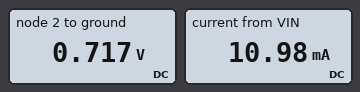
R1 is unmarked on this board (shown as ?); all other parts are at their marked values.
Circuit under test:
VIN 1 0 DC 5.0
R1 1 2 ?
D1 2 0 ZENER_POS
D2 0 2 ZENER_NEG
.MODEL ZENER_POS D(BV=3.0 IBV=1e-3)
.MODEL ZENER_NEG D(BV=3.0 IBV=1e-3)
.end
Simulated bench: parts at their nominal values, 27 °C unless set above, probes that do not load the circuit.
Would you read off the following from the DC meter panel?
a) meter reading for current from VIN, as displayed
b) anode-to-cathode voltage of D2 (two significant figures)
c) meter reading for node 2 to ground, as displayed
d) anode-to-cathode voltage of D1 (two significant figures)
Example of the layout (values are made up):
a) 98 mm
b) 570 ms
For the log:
a) 10.98 mA
b) -720 mV
c) 0.717 V
d) 720 mV
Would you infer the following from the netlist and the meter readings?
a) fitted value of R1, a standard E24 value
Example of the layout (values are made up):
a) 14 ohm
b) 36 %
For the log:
a) 390 Ω
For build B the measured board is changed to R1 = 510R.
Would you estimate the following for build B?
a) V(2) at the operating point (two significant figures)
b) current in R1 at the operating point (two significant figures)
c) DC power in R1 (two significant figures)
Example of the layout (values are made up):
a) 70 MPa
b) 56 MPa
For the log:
a) 710 mV
b) 8.4 mA
c) 36 mW
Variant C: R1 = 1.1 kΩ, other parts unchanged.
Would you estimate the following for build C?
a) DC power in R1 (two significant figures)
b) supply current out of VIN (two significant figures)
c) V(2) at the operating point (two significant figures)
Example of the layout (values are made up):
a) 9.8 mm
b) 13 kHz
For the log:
a) 17 mW
b) 3.9 mA
c) 690 mV
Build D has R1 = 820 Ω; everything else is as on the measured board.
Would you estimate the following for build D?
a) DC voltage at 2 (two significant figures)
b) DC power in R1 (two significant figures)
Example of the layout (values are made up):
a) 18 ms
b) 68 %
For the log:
a) 700 mV
b) 23 mW
